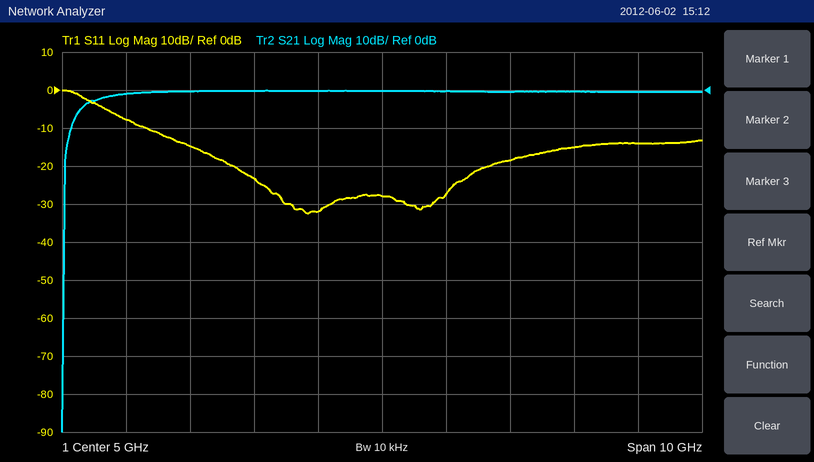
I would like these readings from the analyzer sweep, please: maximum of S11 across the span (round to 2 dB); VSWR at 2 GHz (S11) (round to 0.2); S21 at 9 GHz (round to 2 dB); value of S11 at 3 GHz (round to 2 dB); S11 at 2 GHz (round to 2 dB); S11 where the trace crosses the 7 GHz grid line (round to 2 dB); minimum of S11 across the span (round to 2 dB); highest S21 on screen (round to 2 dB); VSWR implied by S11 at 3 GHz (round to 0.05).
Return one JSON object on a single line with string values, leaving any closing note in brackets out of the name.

{"maximum of S11 across the span": "0 dB", "VSWR at 2 GHz (S11)": "1.4", "S21 at 9 GHz": "0 dB", "value of S11 at 3 GHz": "-24 dB", "S11 at 2 GHz": "-14 dB", "S11 where the trace crosses the 7 GHz grid line": "-18 dB", "minimum of S11 across the span": "-32 dB", "highest S21 on screen": "0 dB", "VSWR implied by S11 at 3 GHz": "1.15"}
